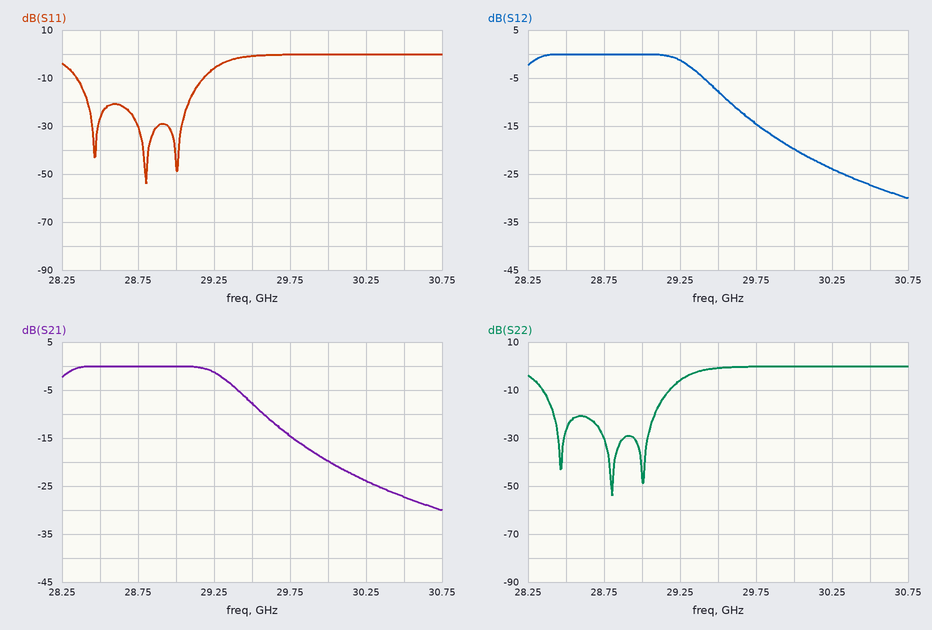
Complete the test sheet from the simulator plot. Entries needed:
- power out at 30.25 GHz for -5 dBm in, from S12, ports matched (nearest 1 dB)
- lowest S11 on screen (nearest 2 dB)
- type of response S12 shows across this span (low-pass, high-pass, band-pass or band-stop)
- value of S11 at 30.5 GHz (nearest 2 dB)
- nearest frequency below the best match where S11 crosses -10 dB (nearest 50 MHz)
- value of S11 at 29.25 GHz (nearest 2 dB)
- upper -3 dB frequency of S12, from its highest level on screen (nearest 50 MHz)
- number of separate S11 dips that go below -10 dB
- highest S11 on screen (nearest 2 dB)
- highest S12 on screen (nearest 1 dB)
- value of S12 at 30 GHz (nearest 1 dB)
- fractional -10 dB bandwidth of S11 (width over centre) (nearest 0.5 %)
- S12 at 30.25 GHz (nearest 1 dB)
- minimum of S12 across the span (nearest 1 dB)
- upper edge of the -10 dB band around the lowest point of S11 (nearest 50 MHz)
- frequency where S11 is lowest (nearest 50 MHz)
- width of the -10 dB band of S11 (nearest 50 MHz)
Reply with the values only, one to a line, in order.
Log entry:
-29 dBm
-54 dB
low-pass
0 dB
28.35 GHz
-6 dB
29.35 GHz
3
0 dB
0 dB
-20 dB
3.0 %
-24 dB
-30 dB
29.20 GHz
28.80 GHz
850 MHz
